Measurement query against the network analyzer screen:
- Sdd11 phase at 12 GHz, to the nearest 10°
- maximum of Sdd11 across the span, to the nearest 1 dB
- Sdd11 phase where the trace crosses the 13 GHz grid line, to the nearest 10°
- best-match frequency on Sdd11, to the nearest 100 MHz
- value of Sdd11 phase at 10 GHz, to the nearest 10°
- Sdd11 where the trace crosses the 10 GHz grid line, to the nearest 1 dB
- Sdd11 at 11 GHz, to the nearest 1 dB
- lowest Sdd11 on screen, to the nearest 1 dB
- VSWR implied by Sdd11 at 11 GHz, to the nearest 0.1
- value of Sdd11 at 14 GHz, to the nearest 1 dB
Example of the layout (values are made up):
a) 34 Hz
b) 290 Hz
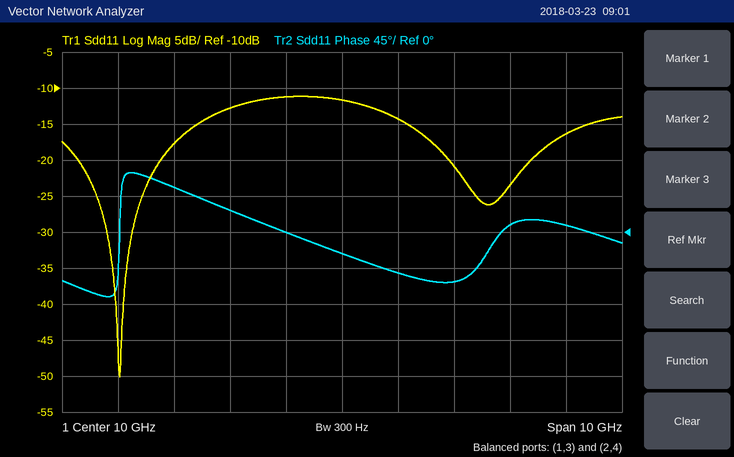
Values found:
a) -60°
b) -11 dB
c) 10°
d) 6.0 GHz
e) -30°
f) -12 dB
g) -14 dB
h) -50 dB
i) 1.5
j) -16 dB
